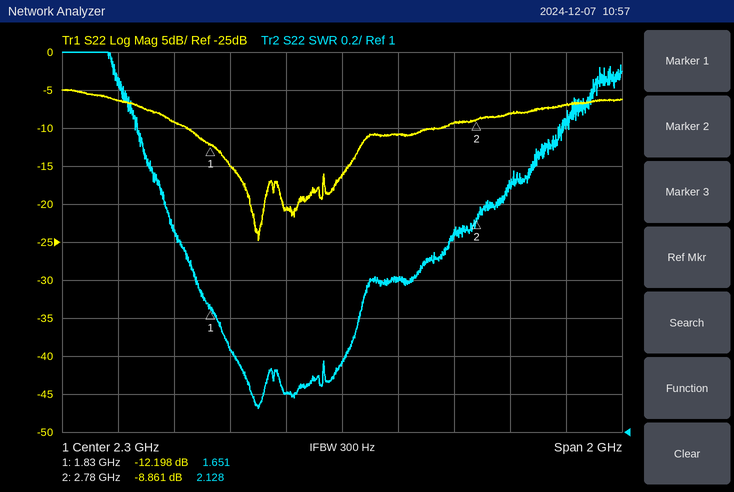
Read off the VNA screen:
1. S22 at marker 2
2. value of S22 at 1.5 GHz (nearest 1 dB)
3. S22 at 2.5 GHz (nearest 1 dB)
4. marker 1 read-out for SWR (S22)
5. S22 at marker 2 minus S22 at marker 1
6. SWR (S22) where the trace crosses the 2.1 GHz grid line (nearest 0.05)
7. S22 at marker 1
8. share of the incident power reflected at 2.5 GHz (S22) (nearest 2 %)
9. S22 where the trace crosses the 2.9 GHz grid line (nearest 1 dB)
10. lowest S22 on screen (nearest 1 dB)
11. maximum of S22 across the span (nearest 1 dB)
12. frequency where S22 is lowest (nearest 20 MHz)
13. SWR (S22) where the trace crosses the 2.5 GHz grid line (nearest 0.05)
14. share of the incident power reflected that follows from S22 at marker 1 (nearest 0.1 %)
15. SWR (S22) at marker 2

-8.861 dB
-6 dB
-11 dB
1.651
3.337 dB
1.20
-12.198 dB
8 %
-8 dB
-25 dB
-5 dB
2.00 GHz
1.80
6.0 %
2.128
